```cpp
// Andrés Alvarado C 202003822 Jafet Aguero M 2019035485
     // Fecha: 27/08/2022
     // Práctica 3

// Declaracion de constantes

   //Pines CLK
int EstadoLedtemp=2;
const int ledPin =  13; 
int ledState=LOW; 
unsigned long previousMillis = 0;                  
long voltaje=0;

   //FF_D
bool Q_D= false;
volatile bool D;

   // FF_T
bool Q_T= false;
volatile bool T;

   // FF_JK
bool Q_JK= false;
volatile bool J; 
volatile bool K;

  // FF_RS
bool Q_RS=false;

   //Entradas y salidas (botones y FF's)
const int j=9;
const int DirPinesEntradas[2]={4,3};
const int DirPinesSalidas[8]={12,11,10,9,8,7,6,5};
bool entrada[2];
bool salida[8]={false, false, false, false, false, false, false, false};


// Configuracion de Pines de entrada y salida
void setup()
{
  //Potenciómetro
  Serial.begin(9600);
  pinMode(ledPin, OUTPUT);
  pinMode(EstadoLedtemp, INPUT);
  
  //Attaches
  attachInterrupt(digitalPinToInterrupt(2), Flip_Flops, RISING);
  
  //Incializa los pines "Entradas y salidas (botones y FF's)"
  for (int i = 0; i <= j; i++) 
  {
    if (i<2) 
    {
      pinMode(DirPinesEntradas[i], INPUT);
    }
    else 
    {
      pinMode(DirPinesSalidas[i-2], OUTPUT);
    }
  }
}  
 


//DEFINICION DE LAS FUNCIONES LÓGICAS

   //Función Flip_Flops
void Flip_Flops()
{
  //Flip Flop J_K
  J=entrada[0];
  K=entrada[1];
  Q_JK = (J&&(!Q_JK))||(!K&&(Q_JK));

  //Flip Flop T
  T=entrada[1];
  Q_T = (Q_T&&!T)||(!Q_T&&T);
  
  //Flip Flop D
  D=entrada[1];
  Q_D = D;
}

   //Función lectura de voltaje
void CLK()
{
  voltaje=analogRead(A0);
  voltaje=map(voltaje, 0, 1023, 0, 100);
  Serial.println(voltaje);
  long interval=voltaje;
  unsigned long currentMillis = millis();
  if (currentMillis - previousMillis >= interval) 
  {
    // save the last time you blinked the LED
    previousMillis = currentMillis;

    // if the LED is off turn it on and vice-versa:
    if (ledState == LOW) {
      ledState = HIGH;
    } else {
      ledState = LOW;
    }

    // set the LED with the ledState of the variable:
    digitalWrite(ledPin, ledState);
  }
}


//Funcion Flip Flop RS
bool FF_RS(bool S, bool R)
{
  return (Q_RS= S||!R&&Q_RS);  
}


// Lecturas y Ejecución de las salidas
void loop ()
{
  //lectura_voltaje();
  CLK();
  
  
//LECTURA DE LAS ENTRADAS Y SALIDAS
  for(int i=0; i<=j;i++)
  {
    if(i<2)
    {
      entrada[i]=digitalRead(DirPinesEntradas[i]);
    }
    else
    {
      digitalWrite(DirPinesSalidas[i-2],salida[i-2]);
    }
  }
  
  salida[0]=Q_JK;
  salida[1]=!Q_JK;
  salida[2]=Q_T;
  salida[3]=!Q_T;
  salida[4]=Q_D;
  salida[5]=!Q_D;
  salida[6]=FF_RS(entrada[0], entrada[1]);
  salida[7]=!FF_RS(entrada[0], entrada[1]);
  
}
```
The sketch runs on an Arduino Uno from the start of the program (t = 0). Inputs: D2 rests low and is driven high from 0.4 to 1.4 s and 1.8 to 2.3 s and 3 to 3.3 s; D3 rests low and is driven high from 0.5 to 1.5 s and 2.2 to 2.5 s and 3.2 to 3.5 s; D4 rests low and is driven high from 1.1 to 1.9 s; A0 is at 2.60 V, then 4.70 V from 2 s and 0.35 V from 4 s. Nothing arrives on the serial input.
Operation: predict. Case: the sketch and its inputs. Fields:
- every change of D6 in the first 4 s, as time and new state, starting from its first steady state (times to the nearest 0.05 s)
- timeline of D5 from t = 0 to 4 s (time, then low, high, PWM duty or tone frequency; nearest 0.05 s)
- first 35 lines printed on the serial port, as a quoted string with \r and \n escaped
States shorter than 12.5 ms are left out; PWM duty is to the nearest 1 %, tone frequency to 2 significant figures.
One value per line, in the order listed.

0 s low; 1.1 s high; 2.2 s low
0 s high; 1.1 s low; 2.2 s high
"52\r\n52\r\n52\r\n52\r\n52\r\n52\r\n52\r\n52\r\n52\r\n52\r\n52\r\n52\r\n52\r\n52\r\n52\r\n52\r\n52\r\n52\r\n52\r\n52\r\n52\r\n52\r\n52\r\n52\r\n52\r\n52\r\n52\r\n52\r\n52\r\n52\r\n52\r\n52\r\n52\r\n52\r\n52\r\n"
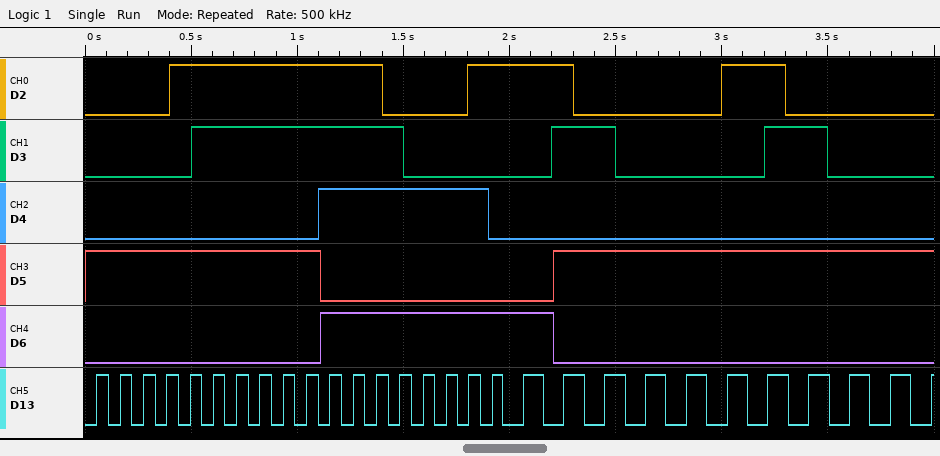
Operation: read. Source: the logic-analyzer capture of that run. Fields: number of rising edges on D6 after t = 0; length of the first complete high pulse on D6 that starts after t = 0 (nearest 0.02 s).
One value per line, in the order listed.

1
1.10 s
